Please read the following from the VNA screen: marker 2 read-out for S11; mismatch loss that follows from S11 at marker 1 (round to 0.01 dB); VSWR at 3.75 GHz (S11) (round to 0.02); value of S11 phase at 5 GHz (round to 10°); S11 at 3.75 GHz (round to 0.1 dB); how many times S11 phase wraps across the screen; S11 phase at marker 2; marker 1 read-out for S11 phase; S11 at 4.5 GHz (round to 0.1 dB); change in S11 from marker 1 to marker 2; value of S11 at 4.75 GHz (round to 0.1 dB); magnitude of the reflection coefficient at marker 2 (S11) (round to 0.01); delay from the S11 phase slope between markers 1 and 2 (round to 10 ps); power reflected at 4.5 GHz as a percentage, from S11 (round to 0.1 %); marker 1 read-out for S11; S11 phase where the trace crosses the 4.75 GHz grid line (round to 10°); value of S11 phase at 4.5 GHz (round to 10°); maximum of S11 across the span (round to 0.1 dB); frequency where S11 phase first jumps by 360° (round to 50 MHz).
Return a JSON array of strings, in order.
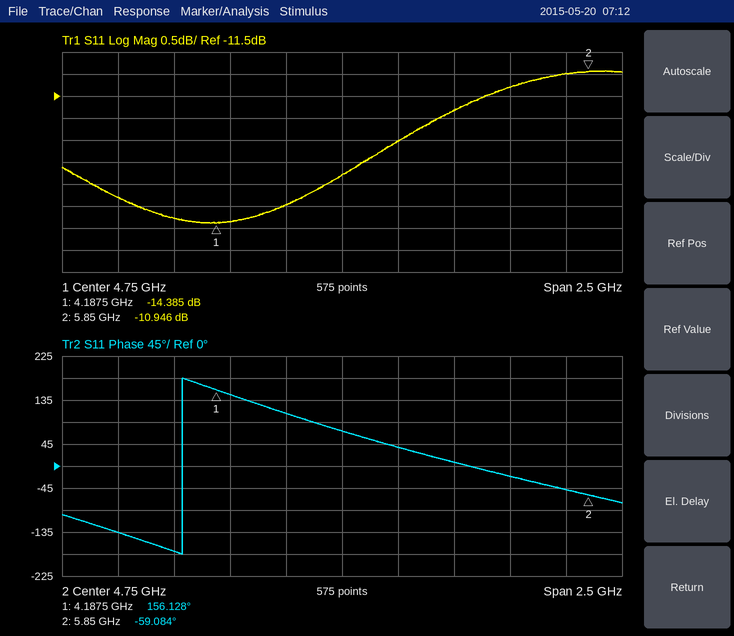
["-10.946 dB", "0.16 dB", "1.52", "40°", "-13.8 dB", "1", "-59.084°", "156.128°", "-14.0 dB", "3.439 dB", "-13.3 dB", "0.28", "360 ps", "4.0 %", "-14.385 dB", "70°", "110°", "-10.9 dB", "4.05 GHz"]
